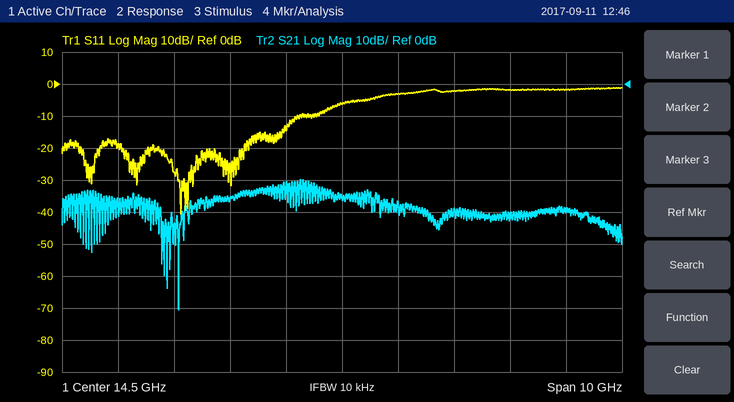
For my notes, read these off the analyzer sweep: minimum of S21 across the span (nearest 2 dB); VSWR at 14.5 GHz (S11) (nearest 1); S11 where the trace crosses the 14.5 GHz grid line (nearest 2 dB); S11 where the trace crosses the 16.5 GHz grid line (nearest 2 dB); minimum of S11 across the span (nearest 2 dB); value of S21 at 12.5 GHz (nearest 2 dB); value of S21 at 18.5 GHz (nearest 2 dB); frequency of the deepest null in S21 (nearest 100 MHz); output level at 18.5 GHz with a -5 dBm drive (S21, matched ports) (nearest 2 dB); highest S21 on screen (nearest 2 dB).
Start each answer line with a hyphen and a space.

- -70 dB
- 3
- -6 dB
- -2 dB
- -40 dB
- -36 dB
- -40 dB
- 11.6 GHz
- -44 dBm
- -30 dB
